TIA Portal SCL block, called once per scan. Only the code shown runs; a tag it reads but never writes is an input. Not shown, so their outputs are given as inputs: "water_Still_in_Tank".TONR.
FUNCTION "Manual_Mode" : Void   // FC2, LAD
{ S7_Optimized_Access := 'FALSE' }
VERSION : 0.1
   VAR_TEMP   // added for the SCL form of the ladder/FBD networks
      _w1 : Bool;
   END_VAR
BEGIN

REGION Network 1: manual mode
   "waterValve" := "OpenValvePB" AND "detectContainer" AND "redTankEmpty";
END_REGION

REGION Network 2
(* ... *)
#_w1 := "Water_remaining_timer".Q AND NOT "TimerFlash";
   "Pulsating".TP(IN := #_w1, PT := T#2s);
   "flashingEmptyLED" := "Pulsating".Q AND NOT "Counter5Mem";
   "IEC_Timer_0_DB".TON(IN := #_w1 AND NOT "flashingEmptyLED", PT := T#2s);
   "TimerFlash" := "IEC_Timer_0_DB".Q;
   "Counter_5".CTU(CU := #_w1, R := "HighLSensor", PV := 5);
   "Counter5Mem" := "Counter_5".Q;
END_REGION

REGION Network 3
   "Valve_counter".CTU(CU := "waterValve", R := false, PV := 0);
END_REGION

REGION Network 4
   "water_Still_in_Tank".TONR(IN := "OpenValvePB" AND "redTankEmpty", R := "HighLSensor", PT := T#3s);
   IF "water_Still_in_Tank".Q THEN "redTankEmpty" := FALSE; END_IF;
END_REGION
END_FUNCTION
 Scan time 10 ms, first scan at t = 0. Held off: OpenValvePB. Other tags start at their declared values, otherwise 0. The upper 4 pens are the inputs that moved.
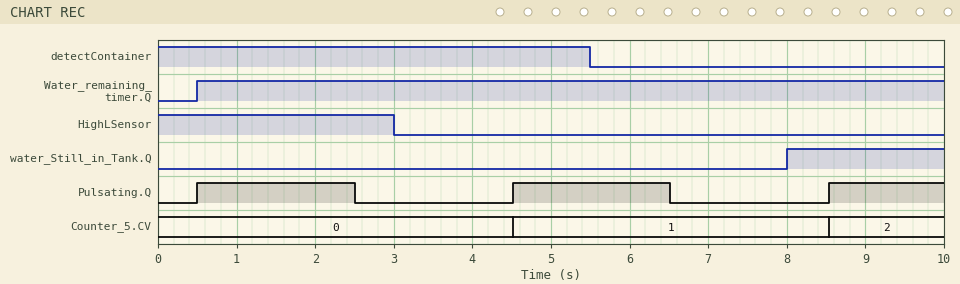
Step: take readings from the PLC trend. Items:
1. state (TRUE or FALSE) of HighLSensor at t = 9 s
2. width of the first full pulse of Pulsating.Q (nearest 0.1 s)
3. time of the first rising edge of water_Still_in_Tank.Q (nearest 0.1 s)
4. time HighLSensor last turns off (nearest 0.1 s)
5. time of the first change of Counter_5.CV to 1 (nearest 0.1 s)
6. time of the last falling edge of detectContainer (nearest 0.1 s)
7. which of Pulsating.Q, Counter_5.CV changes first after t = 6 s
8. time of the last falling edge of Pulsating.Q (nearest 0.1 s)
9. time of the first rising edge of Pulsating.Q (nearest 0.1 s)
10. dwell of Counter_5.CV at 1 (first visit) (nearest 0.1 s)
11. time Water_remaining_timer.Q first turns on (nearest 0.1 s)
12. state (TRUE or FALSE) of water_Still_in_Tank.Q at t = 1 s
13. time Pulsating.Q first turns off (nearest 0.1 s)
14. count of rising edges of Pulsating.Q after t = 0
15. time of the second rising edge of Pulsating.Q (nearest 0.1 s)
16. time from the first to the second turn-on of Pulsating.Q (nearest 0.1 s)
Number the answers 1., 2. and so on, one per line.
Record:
1. FALSE
2. 2.0 s
3. 8.0 s
4. 3.0 s
5. 4.5 s
6. 5.5 s
7. Pulsating.Q
8. 6.5 s
9. 0.5 s
10. 4.0 s
11. 0.5 s
12. FALSE
13. 2.5 s
14. 3
15. 4.5 s
16. 4.0 s
